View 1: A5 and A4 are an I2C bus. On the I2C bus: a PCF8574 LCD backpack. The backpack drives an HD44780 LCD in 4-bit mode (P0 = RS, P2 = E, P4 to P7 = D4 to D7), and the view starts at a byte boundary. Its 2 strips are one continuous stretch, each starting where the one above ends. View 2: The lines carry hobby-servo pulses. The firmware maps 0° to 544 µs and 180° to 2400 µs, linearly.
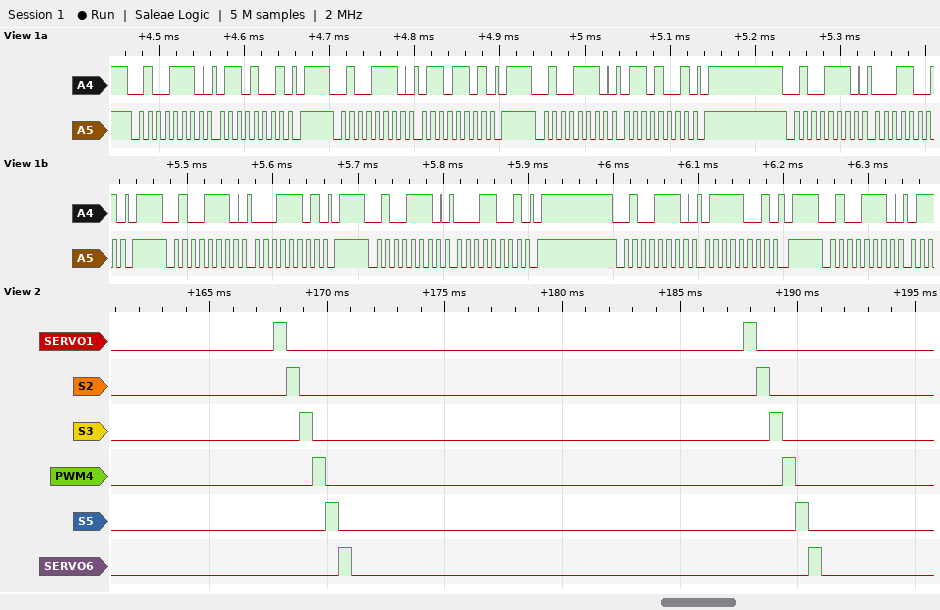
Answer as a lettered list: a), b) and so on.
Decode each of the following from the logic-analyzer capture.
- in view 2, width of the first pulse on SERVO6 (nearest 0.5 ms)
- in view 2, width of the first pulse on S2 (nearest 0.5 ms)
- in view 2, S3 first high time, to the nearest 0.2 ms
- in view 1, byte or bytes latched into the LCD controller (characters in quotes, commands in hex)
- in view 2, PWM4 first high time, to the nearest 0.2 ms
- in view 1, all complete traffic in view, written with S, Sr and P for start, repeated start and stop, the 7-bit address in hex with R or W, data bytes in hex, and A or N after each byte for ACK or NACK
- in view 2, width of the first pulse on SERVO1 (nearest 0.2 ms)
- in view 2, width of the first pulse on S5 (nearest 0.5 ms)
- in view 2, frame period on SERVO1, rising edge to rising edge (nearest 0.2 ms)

a) 0.5 ms
b) 0.5 ms
c) 0.6 ms
d) 'a'
e) 0.6 ms
f) S 27W A 69 A P S 27W A 6D A P S 27W A 69 A P S 27W A 19 A P S 27W A 1D A P S 27W A 19 A P S 27W A 79 A P S 27W A
g) 0.6 ms
h) 0.5 ms
i) 20.0 ms
